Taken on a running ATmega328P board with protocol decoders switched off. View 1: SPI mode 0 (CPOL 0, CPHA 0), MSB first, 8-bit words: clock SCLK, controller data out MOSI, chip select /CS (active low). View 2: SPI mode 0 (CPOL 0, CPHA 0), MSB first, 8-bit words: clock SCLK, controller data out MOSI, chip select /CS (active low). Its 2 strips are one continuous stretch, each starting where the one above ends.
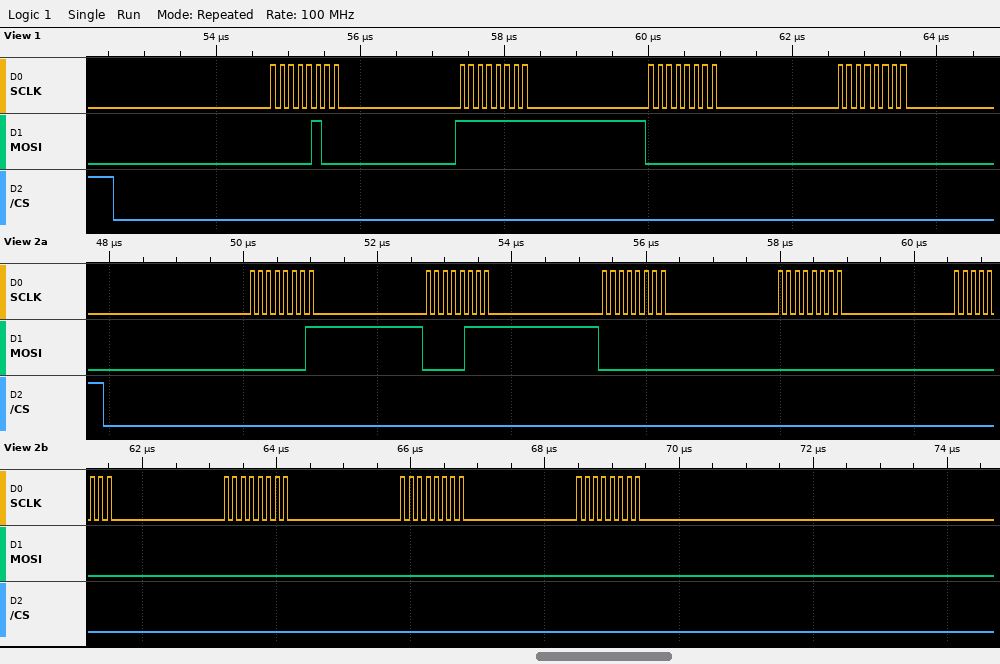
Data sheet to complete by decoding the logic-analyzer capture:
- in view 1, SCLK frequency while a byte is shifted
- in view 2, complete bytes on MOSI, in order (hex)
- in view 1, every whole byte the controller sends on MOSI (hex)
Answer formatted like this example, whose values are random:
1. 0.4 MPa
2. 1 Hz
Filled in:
1. 8 MHz
2. 0x01 0x07 0x00 0x00 0x00 0x00 0x00 0x00
3. 0x04 0xFF 0x00 0x00
